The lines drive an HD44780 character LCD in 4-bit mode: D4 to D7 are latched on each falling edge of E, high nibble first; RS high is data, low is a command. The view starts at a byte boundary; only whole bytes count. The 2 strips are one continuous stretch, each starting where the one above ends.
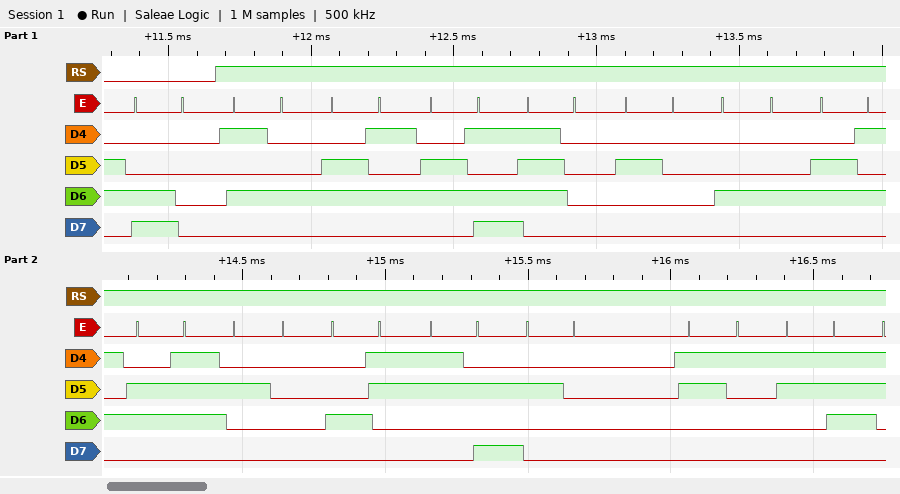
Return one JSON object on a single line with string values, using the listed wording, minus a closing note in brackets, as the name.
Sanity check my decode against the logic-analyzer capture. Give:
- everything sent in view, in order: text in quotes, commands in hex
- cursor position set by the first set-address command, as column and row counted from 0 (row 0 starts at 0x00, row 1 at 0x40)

{"everything sent in view, in order: text in quotes, commands in hex": "0xC0 \"Temp Deg C: 17\"", "cursor position set by the first set-address command, as column and row counted from 0": "column 0, row 1"}
